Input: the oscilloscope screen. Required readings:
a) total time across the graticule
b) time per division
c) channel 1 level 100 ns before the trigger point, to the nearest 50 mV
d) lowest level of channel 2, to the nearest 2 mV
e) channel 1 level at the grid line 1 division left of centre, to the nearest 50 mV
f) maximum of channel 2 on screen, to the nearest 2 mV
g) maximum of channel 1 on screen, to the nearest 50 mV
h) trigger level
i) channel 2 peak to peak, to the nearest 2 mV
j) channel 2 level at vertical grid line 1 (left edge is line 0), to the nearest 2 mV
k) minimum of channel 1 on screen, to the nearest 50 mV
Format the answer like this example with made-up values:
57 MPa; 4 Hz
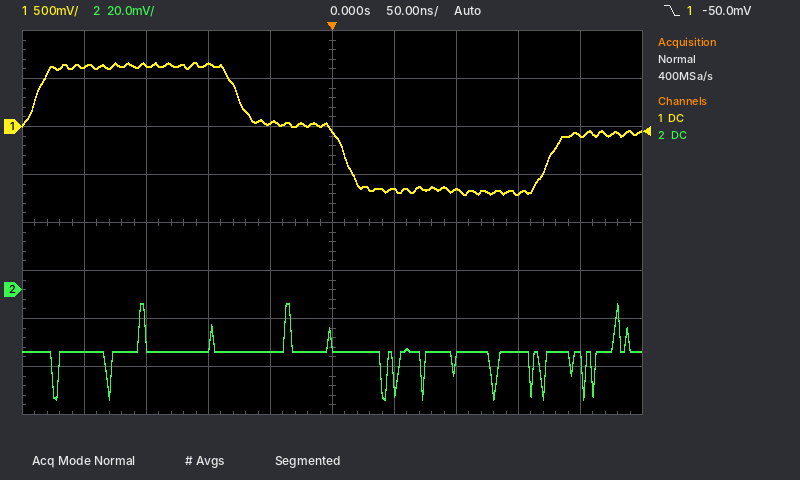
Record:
500 ns; 50 ns; 650 mV; -46 mV; 50 mV; -6 mV; 650 mV; -50.0 mV; 40 mV; -26 mV; -700 mV
